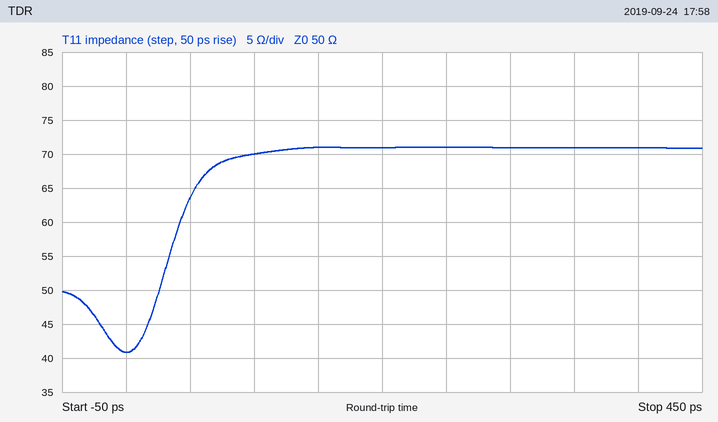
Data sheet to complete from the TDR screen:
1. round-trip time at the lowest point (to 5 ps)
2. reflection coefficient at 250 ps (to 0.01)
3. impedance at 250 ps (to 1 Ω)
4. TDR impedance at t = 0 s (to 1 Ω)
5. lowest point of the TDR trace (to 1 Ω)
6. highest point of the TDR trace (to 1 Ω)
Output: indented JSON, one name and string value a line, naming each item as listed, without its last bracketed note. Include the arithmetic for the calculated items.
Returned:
{
  "round-trip time at the lowest point": "0 ps",
  "reflection coefficient at 250 ps": "(71 − 50)/(71 + 50) ≈ +0.17",
  "impedance at 250 ps": "71 Ω",
  "TDR impedance at t = 0 s": "41 Ω",
  "lowest point of the TDR trace": "41 Ω",
  "highest point of the TDR trace": "71 Ω"
}
